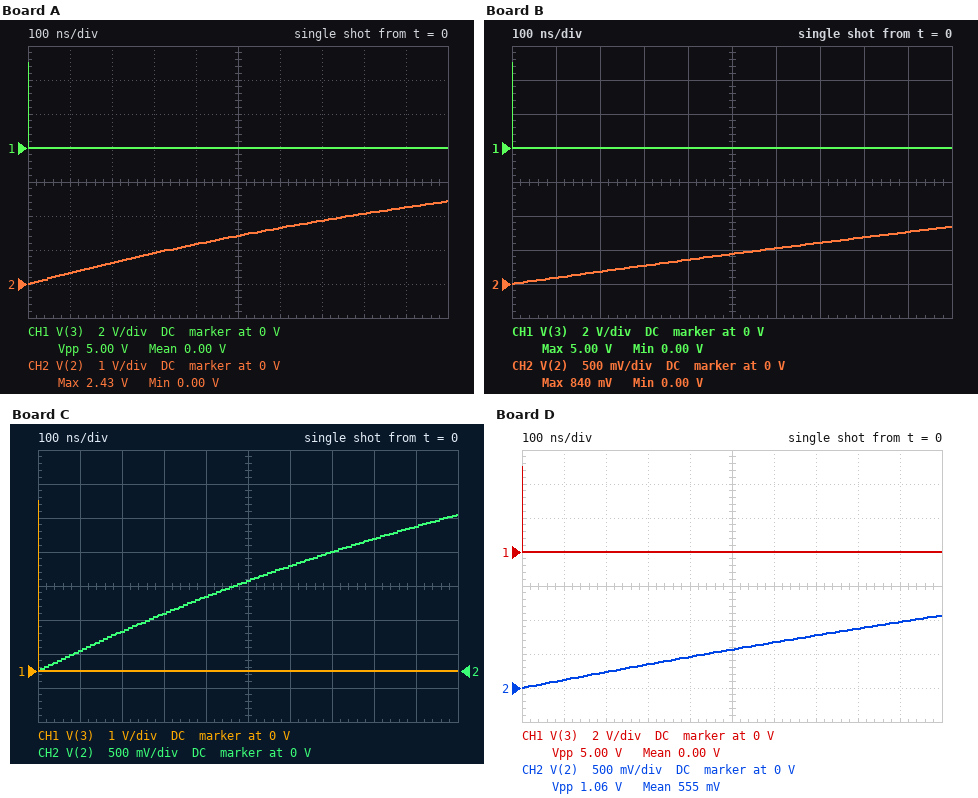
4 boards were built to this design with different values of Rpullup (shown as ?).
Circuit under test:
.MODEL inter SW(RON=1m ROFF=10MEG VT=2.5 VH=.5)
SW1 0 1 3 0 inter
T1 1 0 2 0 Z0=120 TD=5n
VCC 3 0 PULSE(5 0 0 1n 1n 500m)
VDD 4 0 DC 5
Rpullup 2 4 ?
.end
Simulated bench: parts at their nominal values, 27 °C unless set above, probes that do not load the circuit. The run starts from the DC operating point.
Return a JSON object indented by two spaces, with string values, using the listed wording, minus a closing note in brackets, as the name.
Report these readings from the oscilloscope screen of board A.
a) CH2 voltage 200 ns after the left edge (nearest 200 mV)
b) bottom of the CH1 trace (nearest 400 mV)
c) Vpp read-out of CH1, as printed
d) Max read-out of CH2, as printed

{
  "CH2 voltage 200 ns after the left edge": "600 mV",
  "bottom of the CH1 trace": "0 V",
  "Vpp read-out of CH1, as printed": "5.00 V",
  "Max read-out of CH2, as printed": "2.43 V"
}
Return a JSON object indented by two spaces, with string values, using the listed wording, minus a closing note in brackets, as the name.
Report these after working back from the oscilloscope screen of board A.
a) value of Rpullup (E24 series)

{
  "value of Rpullup": "36 kΩ"
}
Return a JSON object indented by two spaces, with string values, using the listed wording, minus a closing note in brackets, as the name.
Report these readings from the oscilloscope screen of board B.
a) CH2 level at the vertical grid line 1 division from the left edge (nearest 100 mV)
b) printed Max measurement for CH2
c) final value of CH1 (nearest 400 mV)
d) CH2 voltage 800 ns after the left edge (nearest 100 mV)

{
  "CH2 level at the vertical grid line 1 division from the left edge": "100 mV",
  "printed Max measurement for CH2": "840 mV",
  "final value of CH1": "0 V",
  "CH2 voltage 800 ns after the left edge": "700 mV"
}
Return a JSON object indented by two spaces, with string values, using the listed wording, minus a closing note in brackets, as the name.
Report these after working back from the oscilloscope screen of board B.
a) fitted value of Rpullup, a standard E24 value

{
  "fitted value of Rpullup, a standard E24 value": "130 kΩ"
}
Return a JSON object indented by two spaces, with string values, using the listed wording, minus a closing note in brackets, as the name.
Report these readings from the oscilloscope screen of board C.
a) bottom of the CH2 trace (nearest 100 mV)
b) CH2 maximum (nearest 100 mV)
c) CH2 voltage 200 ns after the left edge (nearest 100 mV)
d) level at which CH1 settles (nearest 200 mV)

{
  "bottom of the CH2 trace": "0 V",
  "CH2 maximum": "2.3 V",
  "CH2 voltage 200 ns after the left edge": "600 mV",
  "level at which CH1 settles": "0 V"
}
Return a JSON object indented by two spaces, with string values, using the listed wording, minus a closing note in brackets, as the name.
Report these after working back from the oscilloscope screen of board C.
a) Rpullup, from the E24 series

{
  "Rpullup, from the E24 series": "39 kΩ"
}
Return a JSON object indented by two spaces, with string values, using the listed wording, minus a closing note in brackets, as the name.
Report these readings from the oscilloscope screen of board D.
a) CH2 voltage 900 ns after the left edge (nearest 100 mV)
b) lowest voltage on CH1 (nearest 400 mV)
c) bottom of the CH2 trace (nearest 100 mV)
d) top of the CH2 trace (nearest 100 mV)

{
  "CH2 voltage 900 ns after the left edge": "1.0 V",
  "lowest voltage on CH1": "0 V",
  "bottom of the CH2 trace": "0 V",
  "top of the CH2 trace": "1.1 V"
}
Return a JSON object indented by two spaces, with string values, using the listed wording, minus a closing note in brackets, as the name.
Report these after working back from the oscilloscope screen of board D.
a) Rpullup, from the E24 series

{
  "Rpullup, from the E24 series": "100 kΩ"
}
